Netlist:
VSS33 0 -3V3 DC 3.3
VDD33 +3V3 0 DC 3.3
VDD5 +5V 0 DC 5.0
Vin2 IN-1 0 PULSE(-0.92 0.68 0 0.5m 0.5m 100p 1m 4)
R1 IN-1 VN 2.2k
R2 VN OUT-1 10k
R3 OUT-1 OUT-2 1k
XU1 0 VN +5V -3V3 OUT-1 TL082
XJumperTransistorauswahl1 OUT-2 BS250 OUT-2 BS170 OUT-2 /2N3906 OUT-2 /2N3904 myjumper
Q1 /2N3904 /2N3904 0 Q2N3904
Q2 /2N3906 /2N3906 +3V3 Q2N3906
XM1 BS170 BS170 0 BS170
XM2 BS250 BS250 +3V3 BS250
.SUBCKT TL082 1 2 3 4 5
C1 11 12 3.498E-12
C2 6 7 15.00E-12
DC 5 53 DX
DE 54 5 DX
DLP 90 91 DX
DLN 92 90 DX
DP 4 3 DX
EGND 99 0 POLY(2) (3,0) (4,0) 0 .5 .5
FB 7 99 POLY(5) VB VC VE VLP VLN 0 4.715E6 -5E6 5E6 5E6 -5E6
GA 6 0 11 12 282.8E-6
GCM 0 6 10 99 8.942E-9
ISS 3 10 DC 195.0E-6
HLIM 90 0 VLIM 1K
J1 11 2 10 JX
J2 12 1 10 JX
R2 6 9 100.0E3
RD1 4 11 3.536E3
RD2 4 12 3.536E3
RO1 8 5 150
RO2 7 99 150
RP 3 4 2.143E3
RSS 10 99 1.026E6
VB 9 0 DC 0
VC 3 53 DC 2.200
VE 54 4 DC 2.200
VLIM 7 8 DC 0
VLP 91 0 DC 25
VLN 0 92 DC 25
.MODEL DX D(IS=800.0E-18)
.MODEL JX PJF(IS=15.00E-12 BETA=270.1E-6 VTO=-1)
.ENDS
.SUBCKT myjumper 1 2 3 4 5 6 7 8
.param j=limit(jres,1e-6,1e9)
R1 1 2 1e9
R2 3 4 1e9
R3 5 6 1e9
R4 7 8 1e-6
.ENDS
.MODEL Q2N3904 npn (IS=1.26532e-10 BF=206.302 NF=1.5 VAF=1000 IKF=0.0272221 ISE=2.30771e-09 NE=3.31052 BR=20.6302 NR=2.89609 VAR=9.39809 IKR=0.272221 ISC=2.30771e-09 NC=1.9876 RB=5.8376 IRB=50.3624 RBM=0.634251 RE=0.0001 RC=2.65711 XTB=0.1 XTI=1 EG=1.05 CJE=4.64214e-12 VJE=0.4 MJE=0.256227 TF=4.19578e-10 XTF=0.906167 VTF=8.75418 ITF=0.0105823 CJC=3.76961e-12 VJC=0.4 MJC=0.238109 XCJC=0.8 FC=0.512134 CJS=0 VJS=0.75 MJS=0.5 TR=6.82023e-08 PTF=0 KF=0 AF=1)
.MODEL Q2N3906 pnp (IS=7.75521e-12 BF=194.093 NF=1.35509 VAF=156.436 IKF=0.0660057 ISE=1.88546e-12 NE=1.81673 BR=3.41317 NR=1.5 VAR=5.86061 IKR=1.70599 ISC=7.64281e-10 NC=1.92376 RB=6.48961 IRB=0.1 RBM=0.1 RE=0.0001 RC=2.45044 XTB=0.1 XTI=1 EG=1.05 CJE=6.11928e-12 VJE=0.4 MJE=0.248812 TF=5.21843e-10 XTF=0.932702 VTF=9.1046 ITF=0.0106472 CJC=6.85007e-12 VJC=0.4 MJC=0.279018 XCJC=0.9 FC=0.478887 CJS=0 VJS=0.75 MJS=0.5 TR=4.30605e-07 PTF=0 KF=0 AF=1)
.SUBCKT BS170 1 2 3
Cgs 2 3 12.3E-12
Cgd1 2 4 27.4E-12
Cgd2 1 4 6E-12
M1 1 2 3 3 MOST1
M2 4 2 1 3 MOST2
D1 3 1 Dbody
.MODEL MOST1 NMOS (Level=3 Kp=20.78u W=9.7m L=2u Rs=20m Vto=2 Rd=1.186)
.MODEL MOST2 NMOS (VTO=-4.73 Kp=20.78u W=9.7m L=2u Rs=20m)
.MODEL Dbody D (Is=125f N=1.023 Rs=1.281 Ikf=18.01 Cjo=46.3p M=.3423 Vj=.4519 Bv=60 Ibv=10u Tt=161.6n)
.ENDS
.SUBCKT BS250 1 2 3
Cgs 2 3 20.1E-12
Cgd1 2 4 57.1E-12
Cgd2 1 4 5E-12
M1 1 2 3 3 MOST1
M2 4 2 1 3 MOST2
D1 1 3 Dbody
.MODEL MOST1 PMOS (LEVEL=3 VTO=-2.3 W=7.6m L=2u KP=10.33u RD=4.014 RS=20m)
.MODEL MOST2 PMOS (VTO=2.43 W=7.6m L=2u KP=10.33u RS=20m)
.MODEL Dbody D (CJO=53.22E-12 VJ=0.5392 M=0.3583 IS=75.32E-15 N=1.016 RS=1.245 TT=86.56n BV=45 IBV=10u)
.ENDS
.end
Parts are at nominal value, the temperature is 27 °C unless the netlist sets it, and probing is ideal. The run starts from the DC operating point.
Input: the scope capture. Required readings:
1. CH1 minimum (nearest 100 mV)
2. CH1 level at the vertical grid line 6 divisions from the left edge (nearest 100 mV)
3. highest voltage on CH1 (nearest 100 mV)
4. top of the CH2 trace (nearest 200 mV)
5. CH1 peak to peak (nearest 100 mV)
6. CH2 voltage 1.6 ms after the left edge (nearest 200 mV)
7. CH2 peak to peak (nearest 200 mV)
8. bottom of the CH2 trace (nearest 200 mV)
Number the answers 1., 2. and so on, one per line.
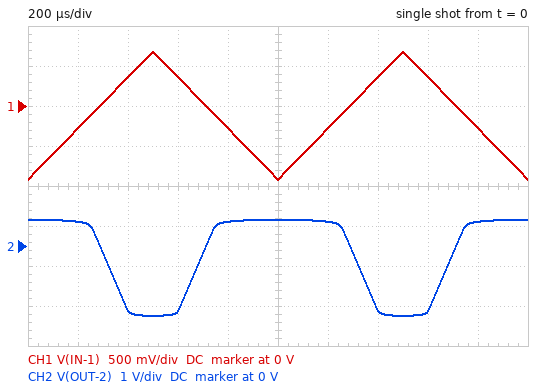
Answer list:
1. -900 mV
2. -300 mV
3. 700 mV
4. 600 mV
5. 1.6 V
6. -1.6 V
7. 2.4 V
8. -1.8 V
